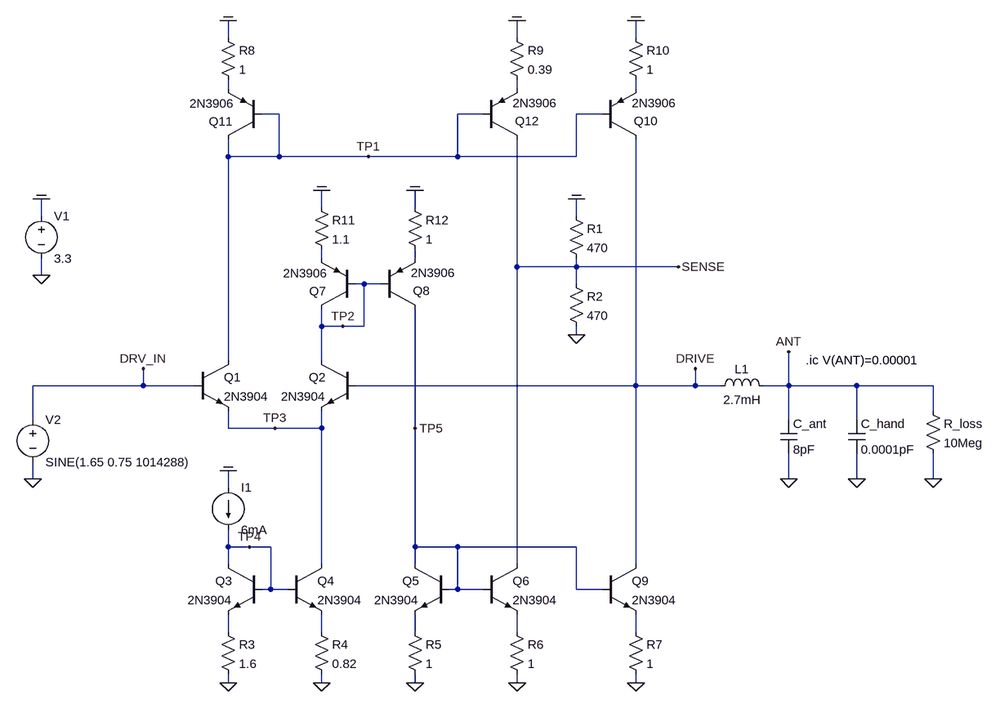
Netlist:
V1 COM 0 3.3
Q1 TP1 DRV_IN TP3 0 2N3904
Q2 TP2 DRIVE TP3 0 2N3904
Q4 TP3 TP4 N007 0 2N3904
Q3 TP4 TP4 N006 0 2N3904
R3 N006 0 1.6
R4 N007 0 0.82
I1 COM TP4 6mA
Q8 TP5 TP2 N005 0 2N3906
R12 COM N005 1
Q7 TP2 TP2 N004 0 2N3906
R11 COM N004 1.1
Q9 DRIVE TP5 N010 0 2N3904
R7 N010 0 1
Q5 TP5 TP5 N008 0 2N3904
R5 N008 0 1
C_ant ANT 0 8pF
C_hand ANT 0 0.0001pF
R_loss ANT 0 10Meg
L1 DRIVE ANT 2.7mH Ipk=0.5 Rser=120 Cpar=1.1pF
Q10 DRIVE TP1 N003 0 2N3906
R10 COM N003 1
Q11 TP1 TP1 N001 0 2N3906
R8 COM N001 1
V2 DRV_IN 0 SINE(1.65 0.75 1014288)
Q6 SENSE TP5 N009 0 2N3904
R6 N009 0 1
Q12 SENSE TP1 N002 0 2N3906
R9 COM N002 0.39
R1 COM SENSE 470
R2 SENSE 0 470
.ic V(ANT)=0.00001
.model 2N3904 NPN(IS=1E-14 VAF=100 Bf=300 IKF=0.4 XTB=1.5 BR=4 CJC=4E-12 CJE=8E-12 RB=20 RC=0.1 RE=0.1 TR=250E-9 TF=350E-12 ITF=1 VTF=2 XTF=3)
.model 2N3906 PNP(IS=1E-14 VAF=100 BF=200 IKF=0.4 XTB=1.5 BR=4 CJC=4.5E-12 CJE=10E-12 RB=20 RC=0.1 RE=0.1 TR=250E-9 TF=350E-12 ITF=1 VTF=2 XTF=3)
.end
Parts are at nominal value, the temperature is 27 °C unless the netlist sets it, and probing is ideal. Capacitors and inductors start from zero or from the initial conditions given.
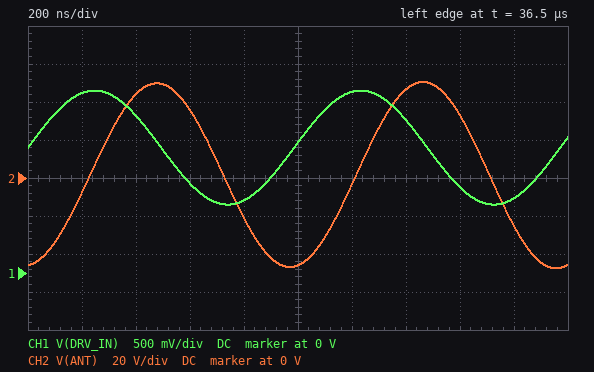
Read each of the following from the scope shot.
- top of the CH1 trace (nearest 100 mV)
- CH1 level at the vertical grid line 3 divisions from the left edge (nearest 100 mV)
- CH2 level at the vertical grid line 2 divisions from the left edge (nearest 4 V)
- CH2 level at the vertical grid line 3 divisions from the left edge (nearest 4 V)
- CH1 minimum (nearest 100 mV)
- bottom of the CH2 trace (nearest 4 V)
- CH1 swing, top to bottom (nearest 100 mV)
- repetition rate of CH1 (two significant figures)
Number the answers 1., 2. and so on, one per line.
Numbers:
1. 2.4 V
2. 1.2 V
3. 44 V
4. 36 V
5. 900 mV
6. -48 V
7. 1.5 V
8. 1.0 MHz
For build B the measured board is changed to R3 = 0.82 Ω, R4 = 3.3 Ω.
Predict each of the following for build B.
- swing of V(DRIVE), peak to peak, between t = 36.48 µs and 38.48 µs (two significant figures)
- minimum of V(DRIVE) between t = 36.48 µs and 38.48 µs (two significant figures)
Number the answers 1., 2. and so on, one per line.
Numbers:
1. 1.4 V
2. 930 mV
